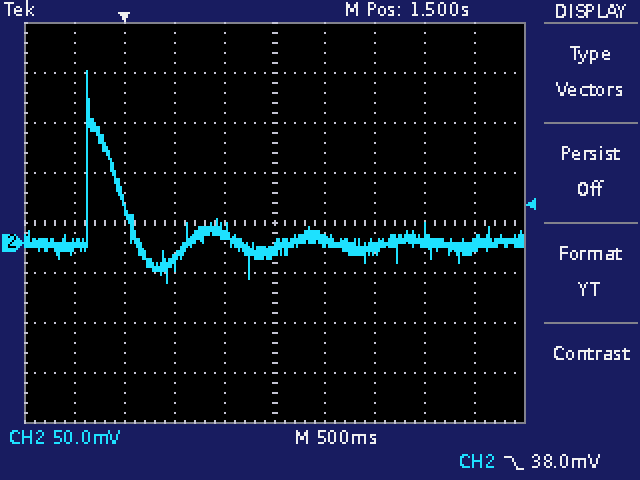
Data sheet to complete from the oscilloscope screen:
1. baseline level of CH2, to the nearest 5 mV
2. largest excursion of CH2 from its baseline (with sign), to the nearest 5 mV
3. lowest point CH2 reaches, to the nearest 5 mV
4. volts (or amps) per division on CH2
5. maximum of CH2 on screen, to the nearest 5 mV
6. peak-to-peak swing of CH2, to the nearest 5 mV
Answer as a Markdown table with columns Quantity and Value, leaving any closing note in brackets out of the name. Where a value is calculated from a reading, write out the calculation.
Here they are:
| Quantity | Value |
|---|---|
| baseline level of CH2, to the nearest 5 mV | 0 mV |
| largest excursion of CH2 from its baseline (with sign), to the nearest 5 mV | 170 mV − (0 mV) = +170 mV |
| lowest point CH2 reaches, to the nearest 5 mV | -40 mV |
| volts (or amps) per division on CH2 | 50 mV |
| maximum of CH2 on screen, to the nearest 5 mV | 170 mV |
| peak-to-peak swing of CH2, to the nearest 5 mV | 170 mV − (-40 mV) = 210 mV |
